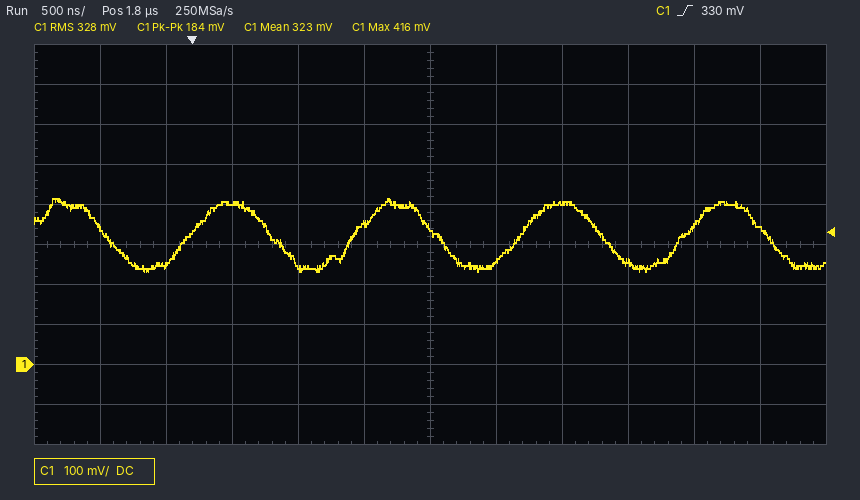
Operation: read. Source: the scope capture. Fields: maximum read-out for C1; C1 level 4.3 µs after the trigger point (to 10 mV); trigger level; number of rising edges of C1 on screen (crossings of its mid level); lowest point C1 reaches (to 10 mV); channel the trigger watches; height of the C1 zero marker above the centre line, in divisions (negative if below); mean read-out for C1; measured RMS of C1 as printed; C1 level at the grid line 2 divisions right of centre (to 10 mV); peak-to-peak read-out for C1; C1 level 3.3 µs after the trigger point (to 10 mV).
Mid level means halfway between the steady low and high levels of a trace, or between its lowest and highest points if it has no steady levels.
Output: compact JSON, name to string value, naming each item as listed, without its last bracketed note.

{"maximum read-out for C1": "416 mV", "C1 level 4.3 µs after the trigger point": "340 mV", "trigger level": "330 mV", "number of rising edges of C1 on screen": "4", "lowest point C1 reaches": "230 mV", "channel the trigger watches": "C1", "height of the C1 zero marker above the centre line, in divisions": "-3.0 div", "mean read-out for C1": "323 mV", "measured RMS of C1 as printed": "328 mV", "C1 level at the grid line 2 divisions right of centre": "400 mV", "peak-to-peak read-out for C1": "184 mV", "C1 level 3.3 µs after the trigger point": "260 mV"}
